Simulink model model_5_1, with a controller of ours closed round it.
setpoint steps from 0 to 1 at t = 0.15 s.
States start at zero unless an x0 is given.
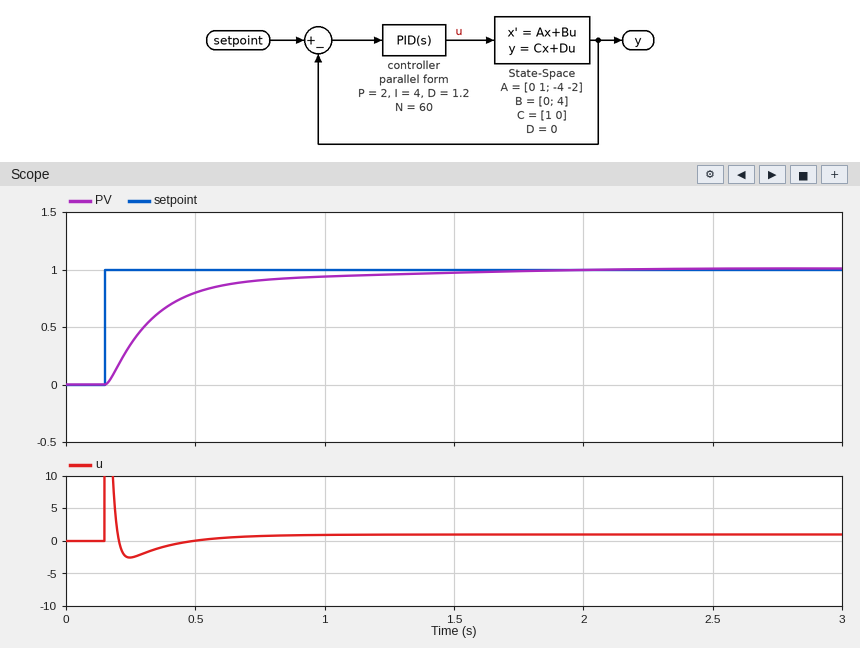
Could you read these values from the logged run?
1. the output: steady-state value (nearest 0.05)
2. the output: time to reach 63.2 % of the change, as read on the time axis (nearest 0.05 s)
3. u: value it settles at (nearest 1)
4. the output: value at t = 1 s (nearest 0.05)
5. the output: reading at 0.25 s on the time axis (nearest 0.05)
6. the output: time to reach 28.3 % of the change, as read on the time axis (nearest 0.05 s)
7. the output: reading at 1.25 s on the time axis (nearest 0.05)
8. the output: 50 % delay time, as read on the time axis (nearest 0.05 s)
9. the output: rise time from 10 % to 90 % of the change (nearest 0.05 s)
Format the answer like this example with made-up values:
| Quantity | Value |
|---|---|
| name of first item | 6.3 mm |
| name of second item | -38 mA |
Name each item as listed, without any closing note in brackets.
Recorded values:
| Quantity | Value |
|---|---|
| the output: steady-state value | 1.00 |
| the output: time to reach 63.2 % of the change, as read on the time axis | 0.35 s |
| u: value it settles at | 1 |
| the output: value at t = 1 s | 0.95 |
| the output: reading at 0.25 s on the time axis | 0.35 |
| the output: time to reach 28.3 % of the change, as read on the time axis | 0.25 s |
| the output: reading at 1.25 s on the time axis | 0.95 |
| the output: 50 % delay time, as read on the time axis | 0.30 s |
| the output: rise time from 10 % to 90 % of the change | 0.55 s |
